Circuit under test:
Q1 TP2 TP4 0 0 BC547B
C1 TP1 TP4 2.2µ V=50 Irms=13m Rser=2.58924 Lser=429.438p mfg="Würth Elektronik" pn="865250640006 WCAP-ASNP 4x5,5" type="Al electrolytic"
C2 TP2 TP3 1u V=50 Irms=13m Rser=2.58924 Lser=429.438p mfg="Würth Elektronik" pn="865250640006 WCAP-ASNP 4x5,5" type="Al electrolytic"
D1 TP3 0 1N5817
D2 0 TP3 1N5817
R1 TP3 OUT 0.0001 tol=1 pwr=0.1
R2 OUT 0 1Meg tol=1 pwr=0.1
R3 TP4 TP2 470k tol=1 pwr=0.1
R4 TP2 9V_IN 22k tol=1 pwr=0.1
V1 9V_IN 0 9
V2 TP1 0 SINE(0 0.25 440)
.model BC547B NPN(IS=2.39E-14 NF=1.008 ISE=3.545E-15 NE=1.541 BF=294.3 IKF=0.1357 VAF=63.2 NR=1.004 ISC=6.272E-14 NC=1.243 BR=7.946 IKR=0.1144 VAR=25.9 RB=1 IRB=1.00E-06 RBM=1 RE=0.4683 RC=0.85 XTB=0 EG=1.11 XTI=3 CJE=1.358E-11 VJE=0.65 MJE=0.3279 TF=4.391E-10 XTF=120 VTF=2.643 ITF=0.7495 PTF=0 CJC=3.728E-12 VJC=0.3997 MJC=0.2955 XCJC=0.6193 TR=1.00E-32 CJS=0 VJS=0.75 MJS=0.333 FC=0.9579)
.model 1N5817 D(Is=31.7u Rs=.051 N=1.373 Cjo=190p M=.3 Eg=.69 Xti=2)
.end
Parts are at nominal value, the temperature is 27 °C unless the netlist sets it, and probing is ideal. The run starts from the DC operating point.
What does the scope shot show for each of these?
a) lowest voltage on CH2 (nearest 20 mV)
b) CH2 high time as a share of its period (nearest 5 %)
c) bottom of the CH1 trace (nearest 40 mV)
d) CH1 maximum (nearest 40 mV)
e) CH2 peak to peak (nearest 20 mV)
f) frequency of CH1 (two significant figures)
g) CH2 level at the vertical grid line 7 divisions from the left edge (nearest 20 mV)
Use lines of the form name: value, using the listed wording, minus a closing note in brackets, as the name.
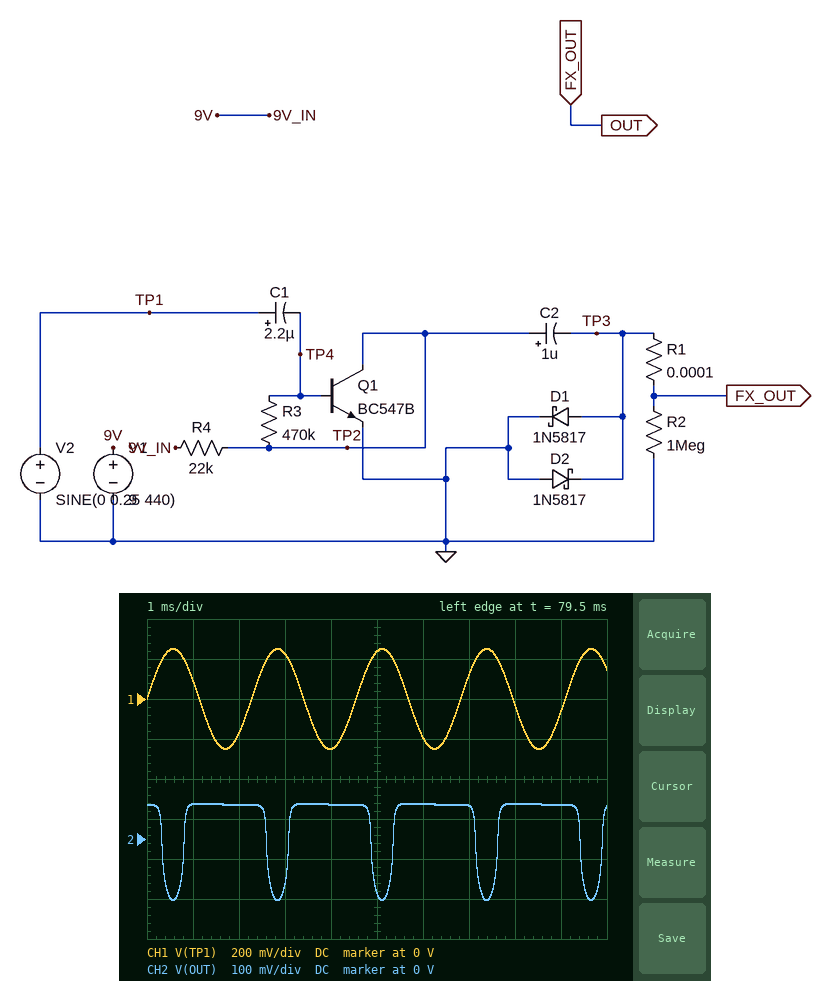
lowest voltage on CH2: -160 mV
CH2 high time as a share of its period: 80 %
bottom of the CH1 trace: -240 mV
CH1 maximum: 240 mV
CH2 peak to peak: 240 mV
frequency of CH1: 440 Hz
CH2 level at the vertical grid line 7 divisions from the left edge: 80 mV
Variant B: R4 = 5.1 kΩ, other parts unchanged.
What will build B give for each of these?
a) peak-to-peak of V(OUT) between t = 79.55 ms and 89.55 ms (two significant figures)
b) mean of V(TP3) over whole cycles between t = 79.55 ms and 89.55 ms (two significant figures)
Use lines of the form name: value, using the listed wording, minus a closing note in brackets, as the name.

peak-to-peak of V(OUT) between t = 79.55 ms and 89.55 ms: 330 mV
mean of V(TP3) over whole cycles between t = 79.55 ms and 89.55 ms: 64 mV
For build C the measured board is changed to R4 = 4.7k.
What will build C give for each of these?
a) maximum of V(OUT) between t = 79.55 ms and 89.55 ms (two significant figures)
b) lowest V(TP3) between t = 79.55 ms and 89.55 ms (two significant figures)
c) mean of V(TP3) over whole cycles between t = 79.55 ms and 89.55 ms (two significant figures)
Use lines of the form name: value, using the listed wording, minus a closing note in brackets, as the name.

maximum of V(OUT) between t = 79.55 ms and 89.55 ms: 140 mV
lowest V(TP3) between t = 79.55 ms and 89.55 ms: -200 mV
mean of V(TP3) over whole cycles between t = 79.55 ms and 89.55 ms: 65 mV
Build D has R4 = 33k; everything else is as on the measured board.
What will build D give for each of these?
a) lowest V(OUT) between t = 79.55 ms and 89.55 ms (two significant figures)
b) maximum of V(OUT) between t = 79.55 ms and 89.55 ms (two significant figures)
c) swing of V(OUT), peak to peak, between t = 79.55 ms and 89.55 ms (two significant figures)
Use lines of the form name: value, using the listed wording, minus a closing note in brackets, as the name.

lowest V(OUT) between t = 79.55 ms and 89.55 ms: -140 mV
maximum of V(OUT) between t = 79.55 ms and 89.55 ms: 74 mV
swing of V(OUT), peak to peak, between t = 79.55 ms and 89.55 ms: 210 mV
